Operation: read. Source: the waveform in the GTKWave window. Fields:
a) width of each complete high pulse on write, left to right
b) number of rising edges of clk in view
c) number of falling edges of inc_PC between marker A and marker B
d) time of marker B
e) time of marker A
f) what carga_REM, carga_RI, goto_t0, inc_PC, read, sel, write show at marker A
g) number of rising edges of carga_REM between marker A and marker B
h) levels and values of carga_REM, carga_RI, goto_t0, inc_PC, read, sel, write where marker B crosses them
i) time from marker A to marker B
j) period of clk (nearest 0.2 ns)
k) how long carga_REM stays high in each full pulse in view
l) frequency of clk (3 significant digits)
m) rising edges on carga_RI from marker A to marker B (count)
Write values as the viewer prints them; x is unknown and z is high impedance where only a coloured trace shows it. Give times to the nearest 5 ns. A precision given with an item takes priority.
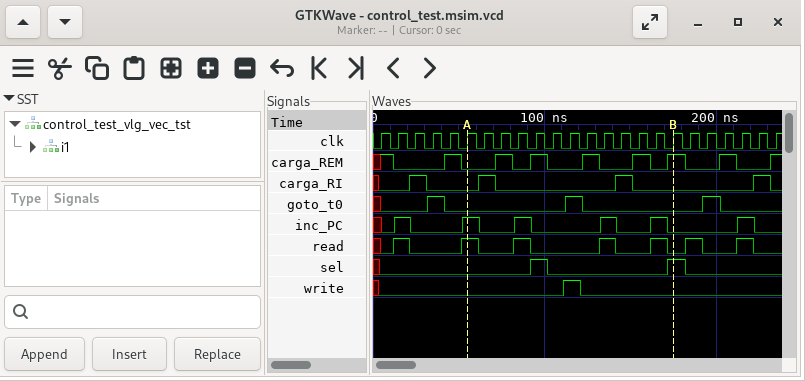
10 ns
24
4
175 ns
55 ns
carga_REM=0, carga_RI=0, goto_t0=0, inc_PC=1, read=1, sel=0, write=0
5
carga_REM=1, carga_RI=0, goto_t0=0, inc_PC=0, read=0, sel=1, write=0
120 ns
10 ns
10 ns, 10 ns, 10 ns, 10 ns, 10 ns, 10 ns, 10 ns
100 MHz
2
